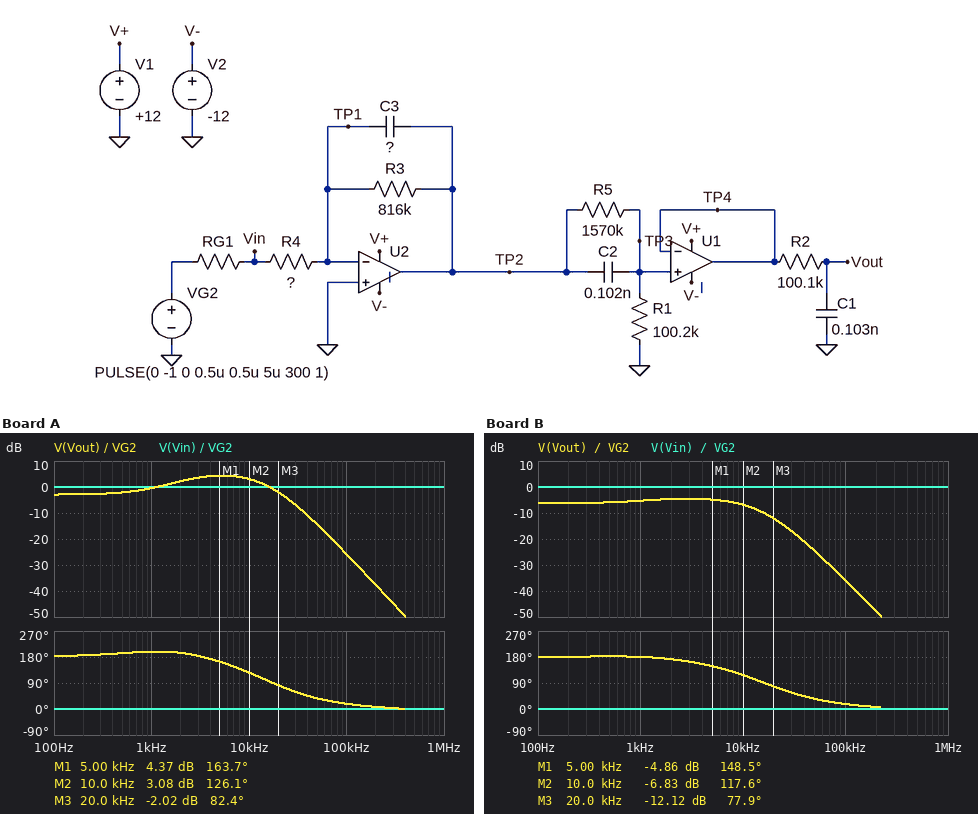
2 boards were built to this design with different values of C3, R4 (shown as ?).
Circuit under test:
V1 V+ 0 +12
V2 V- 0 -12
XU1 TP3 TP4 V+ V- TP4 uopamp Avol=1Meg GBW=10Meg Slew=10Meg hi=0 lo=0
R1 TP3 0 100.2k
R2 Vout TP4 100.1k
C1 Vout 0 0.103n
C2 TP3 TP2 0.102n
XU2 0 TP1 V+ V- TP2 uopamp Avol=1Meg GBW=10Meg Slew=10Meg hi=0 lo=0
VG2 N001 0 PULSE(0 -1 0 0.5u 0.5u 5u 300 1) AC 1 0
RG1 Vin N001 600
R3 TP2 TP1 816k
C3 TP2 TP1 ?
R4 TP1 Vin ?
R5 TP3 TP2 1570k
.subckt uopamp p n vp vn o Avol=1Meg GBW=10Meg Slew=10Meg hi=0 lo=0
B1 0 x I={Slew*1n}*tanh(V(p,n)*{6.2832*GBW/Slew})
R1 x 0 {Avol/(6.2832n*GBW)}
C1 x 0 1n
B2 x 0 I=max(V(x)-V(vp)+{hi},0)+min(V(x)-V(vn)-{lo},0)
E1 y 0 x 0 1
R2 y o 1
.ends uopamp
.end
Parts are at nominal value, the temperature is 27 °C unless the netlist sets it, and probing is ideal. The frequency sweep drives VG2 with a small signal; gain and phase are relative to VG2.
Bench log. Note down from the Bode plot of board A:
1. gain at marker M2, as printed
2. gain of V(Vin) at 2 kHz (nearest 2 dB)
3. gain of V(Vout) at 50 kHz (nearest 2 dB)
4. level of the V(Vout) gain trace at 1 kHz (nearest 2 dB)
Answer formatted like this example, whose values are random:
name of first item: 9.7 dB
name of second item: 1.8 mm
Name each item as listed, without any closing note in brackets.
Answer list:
gain at marker M2, as printed: 3.08 dB
gain of V(Vin) at 2 kHz: 0 dB
gain of V(Vout) at 50 kHz: -14 dB
level of the V(Vout) gain trace at 1 kHz: 0 dB
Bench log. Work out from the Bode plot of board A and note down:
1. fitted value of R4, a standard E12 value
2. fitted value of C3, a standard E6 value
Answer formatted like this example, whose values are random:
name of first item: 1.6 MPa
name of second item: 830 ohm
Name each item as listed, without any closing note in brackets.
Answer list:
fitted value of R4, a standard E12 value: 68 kΩ
fitted value of C3, a standard E6 value: 68 pF
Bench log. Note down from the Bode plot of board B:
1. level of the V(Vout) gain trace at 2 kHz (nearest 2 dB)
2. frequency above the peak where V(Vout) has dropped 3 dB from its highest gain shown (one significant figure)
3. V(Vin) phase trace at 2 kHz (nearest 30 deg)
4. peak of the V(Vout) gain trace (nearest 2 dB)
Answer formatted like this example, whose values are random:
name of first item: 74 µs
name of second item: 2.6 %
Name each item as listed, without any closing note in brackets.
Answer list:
level of the V(Vout) gain trace at 2 kHz: -4 dB
frequency above the peak where V(Vout) has dropped 3 dB from its highest gain shown: 10 kHz
V(Vin) phase trace at 2 kHz: 0 deg
peak of the V(Vout) gain trace: -4 dB
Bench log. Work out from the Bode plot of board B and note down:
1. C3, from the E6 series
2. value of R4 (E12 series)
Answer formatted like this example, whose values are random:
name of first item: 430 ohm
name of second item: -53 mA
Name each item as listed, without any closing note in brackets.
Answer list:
C3, from the E6 series: 150 pF
value of R4: 100 kΩ
